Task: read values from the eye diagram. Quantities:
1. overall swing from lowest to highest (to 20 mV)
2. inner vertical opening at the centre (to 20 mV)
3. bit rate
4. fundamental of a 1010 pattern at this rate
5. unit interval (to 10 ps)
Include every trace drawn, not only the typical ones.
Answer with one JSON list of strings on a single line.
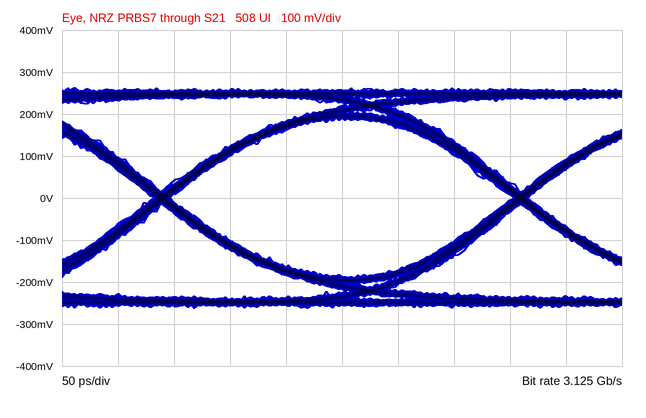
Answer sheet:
["520 mV", "380 mV", "3.125 Gb/s", "1.5625 GHz", "320 ps"]
